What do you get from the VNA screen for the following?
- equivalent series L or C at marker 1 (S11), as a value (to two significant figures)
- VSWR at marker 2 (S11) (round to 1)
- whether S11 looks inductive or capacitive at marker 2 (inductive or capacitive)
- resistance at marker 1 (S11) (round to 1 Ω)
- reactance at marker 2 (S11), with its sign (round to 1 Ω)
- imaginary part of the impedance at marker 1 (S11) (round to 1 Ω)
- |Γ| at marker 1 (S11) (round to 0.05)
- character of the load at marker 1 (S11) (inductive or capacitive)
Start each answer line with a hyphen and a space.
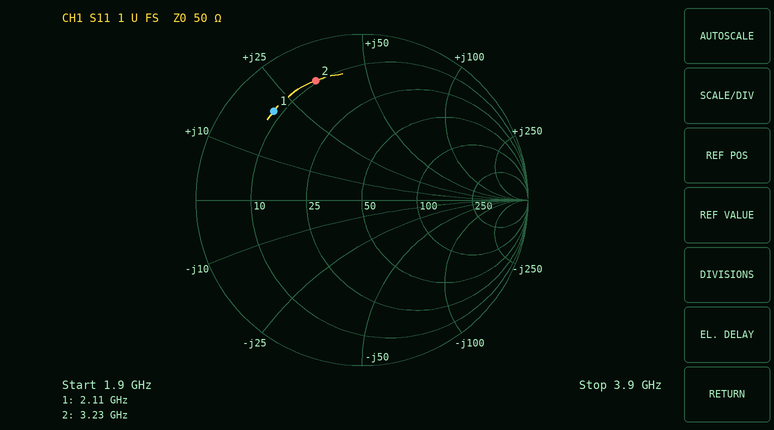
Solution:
- 1.5 nH
- 8
- inductive
- 8 Ω
- +33 Ω
- +20 Ω
- 0.75
- inductive
